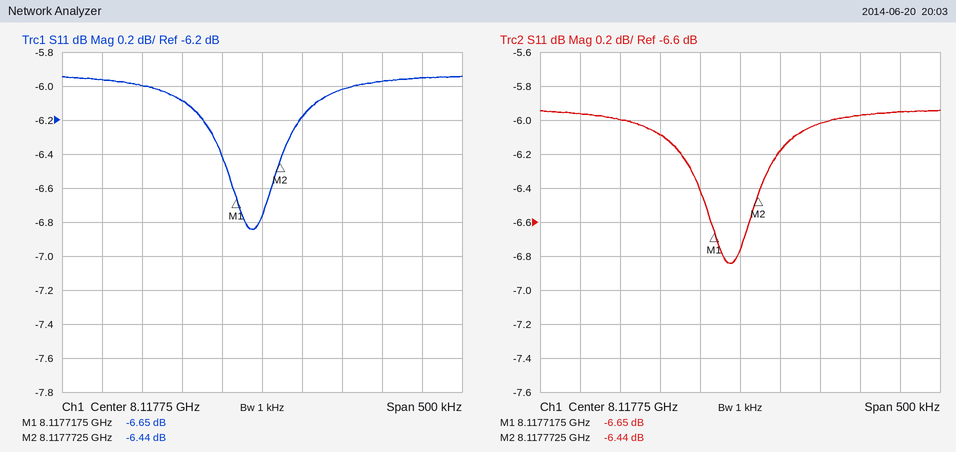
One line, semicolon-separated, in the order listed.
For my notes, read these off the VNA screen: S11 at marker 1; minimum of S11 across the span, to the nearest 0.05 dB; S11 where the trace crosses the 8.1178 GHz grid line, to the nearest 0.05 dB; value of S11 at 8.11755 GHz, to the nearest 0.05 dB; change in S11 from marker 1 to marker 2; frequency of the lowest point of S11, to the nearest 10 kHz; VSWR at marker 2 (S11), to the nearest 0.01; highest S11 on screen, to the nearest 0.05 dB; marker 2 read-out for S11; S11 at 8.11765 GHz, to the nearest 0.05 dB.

-6.65 dB; -6.85 dB; -6.20 dB; -5.95 dB; 0.21 dB; 8.11774 GHz; 2.82; -5.95 dB; -6.44 dB; -6.10 dB
